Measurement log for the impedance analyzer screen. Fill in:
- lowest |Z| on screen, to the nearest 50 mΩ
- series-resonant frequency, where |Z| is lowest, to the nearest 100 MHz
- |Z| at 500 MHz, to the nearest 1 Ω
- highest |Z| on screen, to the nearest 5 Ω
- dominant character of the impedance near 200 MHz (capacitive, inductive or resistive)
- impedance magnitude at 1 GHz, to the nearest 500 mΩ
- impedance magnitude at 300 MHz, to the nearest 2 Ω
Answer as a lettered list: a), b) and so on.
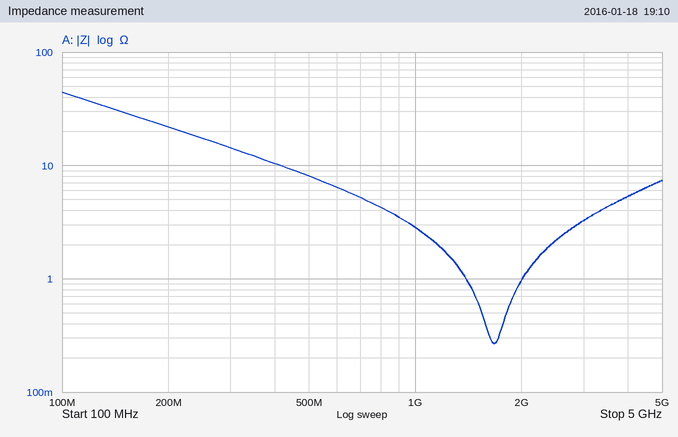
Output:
a) 250 mΩ
b) 1.7 GHz
c) 8 Ω
d) 45 Ω
e) capacitive
f) 3.0 Ω
g) 14 Ω
